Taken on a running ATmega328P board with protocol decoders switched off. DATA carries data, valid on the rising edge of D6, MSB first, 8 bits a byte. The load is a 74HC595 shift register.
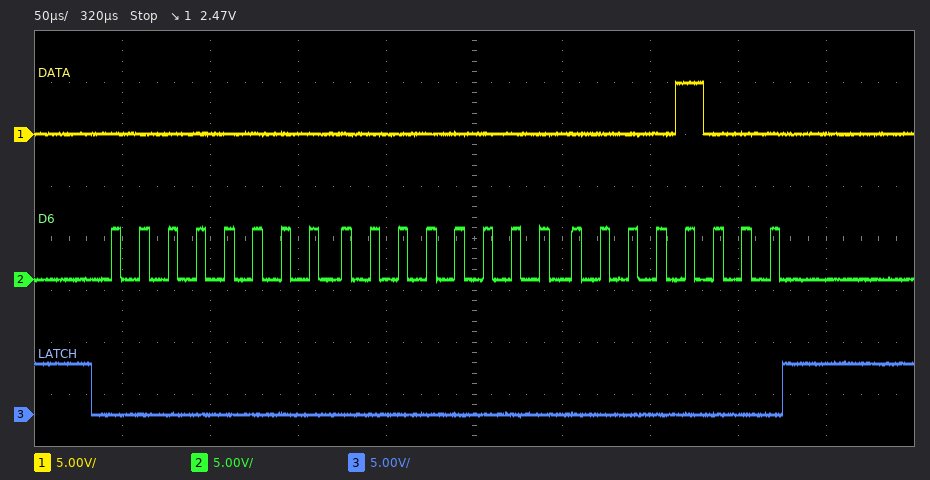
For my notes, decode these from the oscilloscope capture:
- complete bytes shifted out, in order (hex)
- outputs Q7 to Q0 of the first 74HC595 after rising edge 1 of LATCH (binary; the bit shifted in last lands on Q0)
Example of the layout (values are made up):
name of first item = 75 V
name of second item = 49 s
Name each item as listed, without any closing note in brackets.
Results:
complete bytes shifted out, in order = 00 00 08
outputs Q7 to Q0 of the first 74HC595 after rising edge 1 of LATCH = 00001000
